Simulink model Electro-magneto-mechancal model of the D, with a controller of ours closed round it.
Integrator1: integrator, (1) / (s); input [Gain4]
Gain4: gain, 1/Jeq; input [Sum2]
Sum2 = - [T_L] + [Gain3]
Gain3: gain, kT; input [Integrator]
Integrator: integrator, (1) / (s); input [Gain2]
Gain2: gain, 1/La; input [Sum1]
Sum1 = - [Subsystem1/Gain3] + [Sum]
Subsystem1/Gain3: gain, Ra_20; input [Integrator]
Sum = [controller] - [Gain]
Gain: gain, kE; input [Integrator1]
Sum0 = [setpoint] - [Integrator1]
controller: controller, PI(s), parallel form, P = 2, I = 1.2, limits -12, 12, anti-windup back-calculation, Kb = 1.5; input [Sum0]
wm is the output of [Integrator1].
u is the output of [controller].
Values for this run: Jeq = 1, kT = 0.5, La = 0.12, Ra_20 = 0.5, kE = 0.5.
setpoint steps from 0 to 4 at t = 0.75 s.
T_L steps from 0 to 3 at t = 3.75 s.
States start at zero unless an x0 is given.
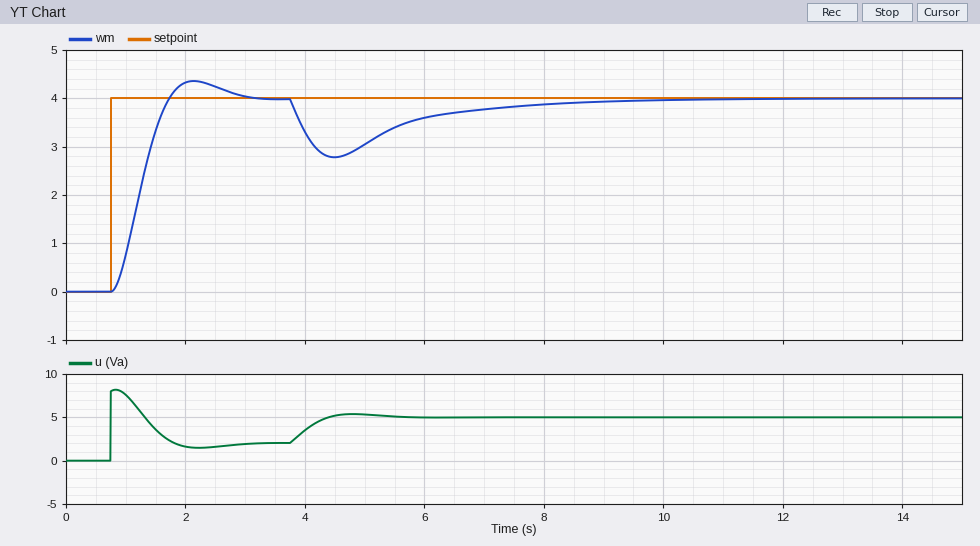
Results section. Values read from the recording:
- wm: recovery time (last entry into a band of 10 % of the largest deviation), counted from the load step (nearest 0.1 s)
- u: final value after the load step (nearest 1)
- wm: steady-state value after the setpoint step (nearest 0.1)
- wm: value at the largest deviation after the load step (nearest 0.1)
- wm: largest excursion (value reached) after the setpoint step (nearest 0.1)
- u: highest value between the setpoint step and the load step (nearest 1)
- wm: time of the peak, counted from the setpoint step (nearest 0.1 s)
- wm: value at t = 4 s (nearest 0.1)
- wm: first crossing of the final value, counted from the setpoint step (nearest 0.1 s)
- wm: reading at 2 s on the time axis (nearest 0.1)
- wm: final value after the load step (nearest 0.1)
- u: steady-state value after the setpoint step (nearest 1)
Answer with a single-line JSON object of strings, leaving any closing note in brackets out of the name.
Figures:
{"wm: recovery time (last entry into a band of 10 % of the largest deviation), counted from the load step": "4.3 s", "u: final value after the load step": "5", "wm: steady-state value after the setpoint step": "4.0", "wm: value at the largest deviation after the load step": "2.8", "wm: largest excursion (value reached) after the setpoint step": "4.4", "u: highest value between the setpoint step and the load step": "8", "wm: time of the peak, counted from the setpoint step": "1.4 s", "wm: value at t = 4 s": "3.3", "wm: first crossing of the final value, counted from the setpoint step": "1.0 s", "wm: reading at 2 s on the time axis": "4.3", "wm: final value after the load step": "4.0", "u: steady-state value after the setpoint step": "2"}
